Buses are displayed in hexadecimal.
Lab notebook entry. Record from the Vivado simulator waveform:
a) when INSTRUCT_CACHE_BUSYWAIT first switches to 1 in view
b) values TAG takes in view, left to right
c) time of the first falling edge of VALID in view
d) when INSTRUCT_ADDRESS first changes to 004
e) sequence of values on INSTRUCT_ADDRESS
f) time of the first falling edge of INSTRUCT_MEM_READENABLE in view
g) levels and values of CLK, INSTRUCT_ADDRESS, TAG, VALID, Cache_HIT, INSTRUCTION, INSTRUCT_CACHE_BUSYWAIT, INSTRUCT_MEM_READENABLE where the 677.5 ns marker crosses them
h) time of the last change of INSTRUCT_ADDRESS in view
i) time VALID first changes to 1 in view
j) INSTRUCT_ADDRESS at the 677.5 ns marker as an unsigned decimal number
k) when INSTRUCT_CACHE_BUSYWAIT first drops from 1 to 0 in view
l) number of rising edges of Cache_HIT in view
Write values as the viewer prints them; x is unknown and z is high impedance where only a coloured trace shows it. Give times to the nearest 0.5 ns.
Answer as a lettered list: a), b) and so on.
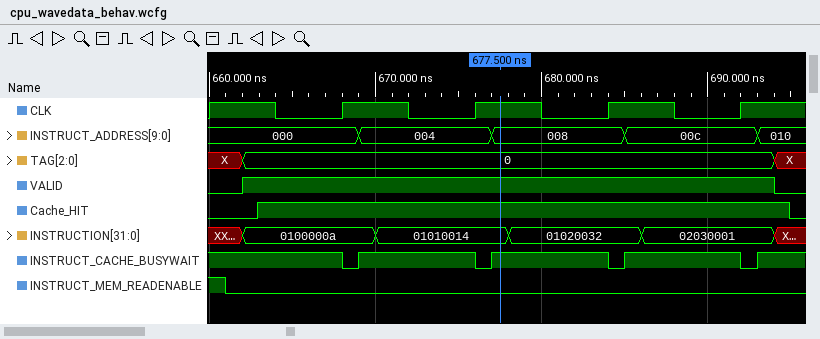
a) 669 ns
b) X, 0, X
c) 694 ns
d) 669 ns
e) 000, 004, 008, 00c, 010
f) 661 ns
g) CLK=1, INSTRUCT_ADDRESS=008, TAG=0, VALID=1, Cache_HIT=1, INSTRUCTION=01010014, INSTRUCT_CACHE_BUSYWAIT=1, INSTRUCT_MEM_READENABLE=0
h) 693 ns
i) 662 ns
j) 8
k) 668 ns
l) 1
